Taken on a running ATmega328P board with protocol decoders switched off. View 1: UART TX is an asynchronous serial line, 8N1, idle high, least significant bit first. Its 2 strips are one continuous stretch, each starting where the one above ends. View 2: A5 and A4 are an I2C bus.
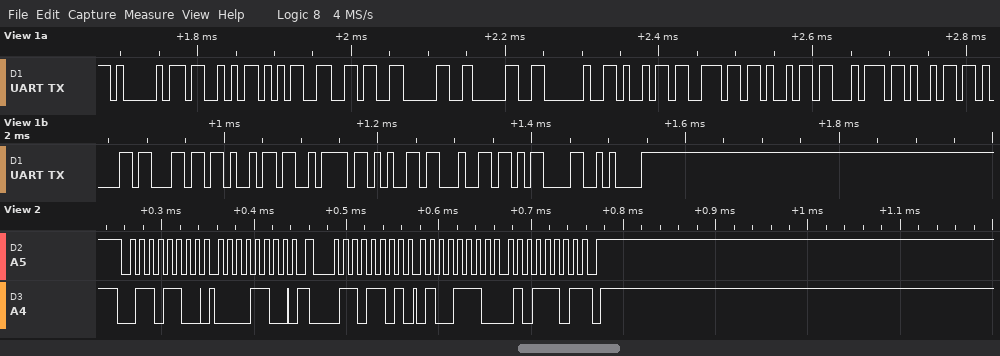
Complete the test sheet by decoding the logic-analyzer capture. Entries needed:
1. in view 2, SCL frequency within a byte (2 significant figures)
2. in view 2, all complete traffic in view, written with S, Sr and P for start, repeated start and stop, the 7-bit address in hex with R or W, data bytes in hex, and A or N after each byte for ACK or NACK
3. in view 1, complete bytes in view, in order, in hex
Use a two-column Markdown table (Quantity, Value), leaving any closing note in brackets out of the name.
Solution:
| Quantity | Value |
|---|---|
| in view 2, SCL frequency within a byte | 100 kHz |
| in view 2, all complete traffic in view, written with S, Sr and P for start, repeated start and stop, the 7-bit address in hex with R or W, data bytes in hex, and A or N after each byte for ACK or NACK | S 36W A 0C A Sr 36R A 4E A 5D N P |
| in view 1, complete bytes in view, in order, in hex | 41 53 35 36 30 30 20 69 6E 69 74 69 61 6C 69 7A 65 64 0D 0A |
